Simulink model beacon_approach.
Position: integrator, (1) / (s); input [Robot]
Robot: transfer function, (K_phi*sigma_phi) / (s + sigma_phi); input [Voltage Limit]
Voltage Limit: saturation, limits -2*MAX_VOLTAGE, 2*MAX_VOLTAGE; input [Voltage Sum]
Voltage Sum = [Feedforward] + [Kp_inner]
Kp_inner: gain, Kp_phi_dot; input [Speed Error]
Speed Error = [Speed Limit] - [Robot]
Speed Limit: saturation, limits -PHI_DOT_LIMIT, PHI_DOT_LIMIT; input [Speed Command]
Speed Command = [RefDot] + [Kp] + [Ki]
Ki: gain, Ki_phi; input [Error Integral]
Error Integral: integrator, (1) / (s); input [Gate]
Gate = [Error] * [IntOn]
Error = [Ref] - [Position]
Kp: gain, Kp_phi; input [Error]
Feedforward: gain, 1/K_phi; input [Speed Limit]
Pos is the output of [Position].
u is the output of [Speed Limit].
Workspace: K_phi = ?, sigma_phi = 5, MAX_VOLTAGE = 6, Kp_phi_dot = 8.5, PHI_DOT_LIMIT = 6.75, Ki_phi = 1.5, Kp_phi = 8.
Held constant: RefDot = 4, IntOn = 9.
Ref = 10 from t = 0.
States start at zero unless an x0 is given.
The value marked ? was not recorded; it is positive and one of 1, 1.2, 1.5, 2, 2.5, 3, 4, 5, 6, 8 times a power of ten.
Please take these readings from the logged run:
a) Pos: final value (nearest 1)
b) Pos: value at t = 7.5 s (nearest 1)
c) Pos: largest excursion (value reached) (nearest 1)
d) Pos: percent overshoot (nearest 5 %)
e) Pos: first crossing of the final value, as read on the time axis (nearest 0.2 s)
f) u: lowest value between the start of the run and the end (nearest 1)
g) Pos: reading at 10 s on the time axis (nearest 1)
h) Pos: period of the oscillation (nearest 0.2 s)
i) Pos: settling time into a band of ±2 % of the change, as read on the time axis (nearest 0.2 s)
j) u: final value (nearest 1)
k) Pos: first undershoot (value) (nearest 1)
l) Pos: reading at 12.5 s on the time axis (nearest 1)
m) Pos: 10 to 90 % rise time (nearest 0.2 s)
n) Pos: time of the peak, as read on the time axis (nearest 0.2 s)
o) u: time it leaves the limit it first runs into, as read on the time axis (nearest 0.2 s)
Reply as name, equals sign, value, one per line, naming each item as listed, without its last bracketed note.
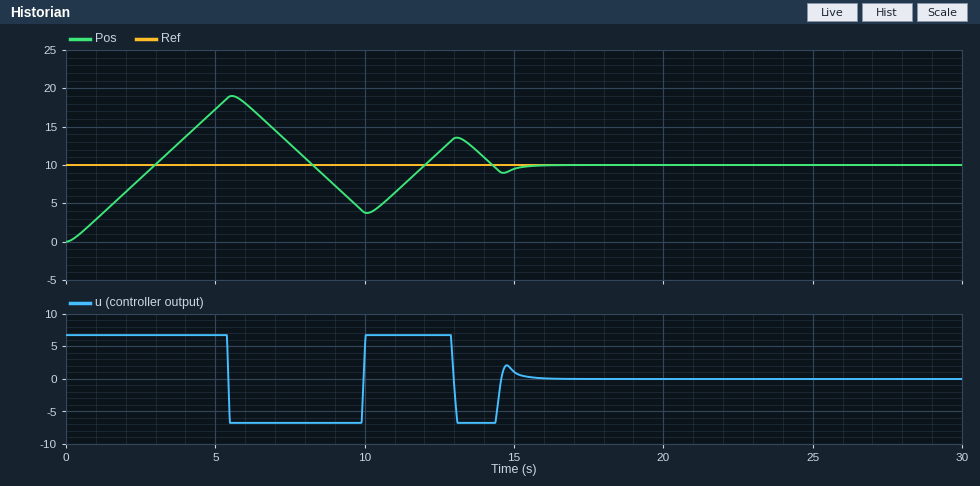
Pos: final value = 10
Pos: value at t = 7.5 s = 13
Pos: largest excursion (value reached) = 19
Pos: percent overshoot = 90 %
Pos: first crossing of the final value, as read on the time axis = 3.0 s
u: lowest value between the start of the run and the end = -7
Pos: reading at 10 s on the time axis = 4
Pos: period of the oscillation = 7.6 s
Pos: settling time into a band of ±2 % of the change, as read on the time axis = 15.4 s
u: final value = 0
Pos: first undershoot (value) = 4
Pos: reading at 12.5 s on the time axis = 12
Pos: 10 to 90 % rise time = 2.2 s
Pos: time of the peak, as read on the time axis = 5.6 s
u: time it leaves the limit it first runs into, as read on the time axis = 5.4 s
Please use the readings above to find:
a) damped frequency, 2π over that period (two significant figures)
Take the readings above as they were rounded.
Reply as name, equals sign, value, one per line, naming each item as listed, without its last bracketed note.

damped frequency, 2π over that period = 0.83 rad/s
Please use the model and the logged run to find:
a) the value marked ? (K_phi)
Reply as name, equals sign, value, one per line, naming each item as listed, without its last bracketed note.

the value marked ? = 0.3
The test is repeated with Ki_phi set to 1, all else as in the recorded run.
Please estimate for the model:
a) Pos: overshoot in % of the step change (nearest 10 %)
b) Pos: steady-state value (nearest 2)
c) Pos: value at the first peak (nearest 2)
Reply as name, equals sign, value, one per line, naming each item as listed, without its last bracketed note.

Pos: overshoot in % of the step change = 80 %
Pos: steady-state value = 10
Pos: value at the first peak = 18
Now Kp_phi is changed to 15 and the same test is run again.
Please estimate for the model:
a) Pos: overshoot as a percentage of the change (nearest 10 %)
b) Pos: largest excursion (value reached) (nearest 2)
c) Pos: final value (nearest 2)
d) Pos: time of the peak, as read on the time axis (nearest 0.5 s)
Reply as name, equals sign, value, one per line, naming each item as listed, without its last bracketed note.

Pos: overshoot as a percentage of the change = 80 %
Pos: largest excursion (value reached) = 18
Pos: final value = 10
Pos: time of the peak, as read on the time axis = 5.0 s
